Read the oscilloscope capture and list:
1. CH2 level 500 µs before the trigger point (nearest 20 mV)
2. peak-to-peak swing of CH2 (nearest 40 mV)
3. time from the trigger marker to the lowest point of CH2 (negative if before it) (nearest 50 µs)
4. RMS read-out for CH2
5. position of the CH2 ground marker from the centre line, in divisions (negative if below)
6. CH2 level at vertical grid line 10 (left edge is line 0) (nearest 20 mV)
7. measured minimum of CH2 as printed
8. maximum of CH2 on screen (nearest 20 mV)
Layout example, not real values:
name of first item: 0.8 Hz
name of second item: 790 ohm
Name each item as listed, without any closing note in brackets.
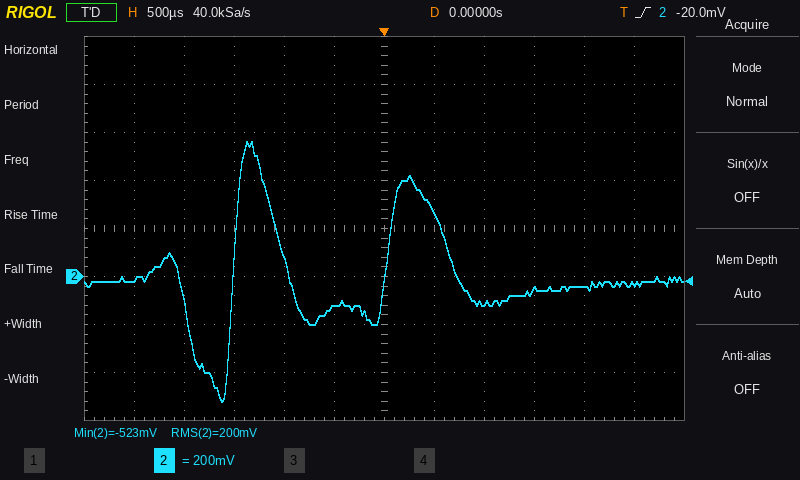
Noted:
CH2 level 500 µs before the trigger point: -120 mV
peak-to-peak swing of CH2: 1.08 V
time from the trigger marker to the lowest point of CH2 (negative if before it): -1.60 ms
RMS read-out for CH2: 200 mV
position of the CH2 ground marker from the centre line, in divisions: -1.0 div
CH2 level at vertical grid line 10 (left edge is line 0): -40 mV
measured minimum of CH2 as printed: -523 mV
maximum of CH2 on screen: 560 mV
